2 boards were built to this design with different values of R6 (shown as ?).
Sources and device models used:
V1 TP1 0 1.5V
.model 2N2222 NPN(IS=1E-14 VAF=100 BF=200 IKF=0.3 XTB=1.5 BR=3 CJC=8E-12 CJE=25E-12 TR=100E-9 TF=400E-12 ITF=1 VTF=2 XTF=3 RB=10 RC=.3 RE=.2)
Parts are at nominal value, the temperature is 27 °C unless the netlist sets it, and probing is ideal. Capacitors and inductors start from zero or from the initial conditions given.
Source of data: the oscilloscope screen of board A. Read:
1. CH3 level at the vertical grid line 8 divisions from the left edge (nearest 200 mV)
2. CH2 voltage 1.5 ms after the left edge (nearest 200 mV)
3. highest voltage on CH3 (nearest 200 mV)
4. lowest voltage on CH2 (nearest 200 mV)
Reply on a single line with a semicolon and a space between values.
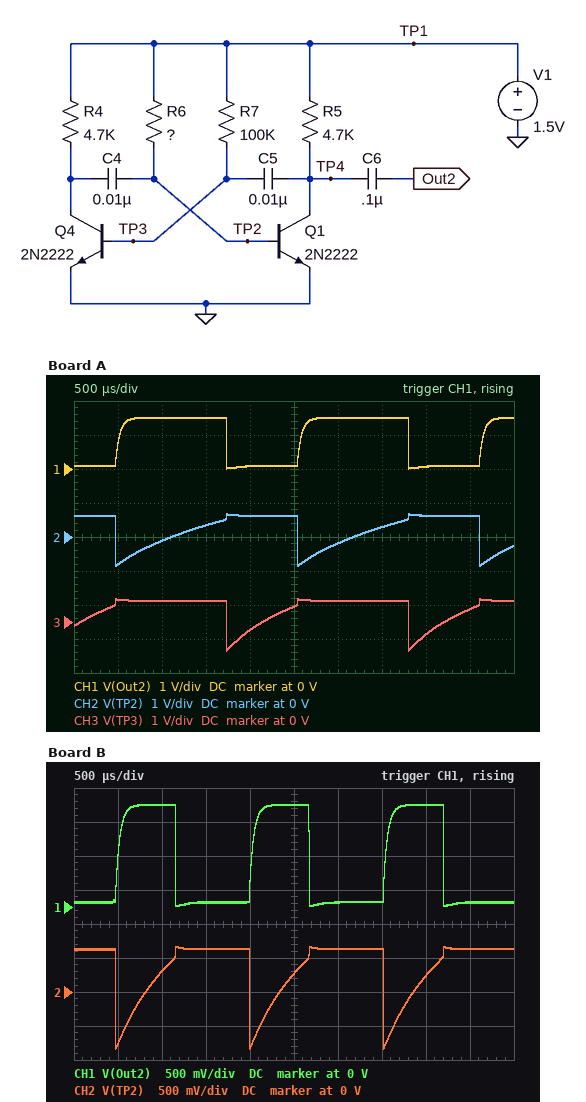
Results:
-400 mV; 400 mV; 600 mV; -800 mV
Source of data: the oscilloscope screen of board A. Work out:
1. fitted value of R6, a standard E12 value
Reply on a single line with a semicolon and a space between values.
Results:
150 kΩ
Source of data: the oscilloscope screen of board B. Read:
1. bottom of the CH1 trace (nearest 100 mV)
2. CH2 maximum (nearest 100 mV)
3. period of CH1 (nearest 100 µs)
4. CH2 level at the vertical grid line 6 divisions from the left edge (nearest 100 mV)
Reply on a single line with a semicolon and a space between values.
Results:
0 V; 700 mV; 1.5 ms; 600 mV
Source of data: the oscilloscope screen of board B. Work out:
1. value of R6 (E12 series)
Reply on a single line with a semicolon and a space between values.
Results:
82 kΩ
